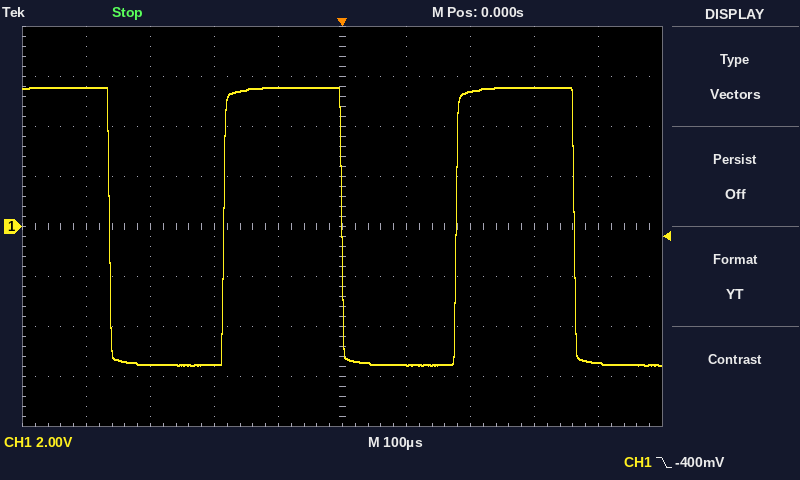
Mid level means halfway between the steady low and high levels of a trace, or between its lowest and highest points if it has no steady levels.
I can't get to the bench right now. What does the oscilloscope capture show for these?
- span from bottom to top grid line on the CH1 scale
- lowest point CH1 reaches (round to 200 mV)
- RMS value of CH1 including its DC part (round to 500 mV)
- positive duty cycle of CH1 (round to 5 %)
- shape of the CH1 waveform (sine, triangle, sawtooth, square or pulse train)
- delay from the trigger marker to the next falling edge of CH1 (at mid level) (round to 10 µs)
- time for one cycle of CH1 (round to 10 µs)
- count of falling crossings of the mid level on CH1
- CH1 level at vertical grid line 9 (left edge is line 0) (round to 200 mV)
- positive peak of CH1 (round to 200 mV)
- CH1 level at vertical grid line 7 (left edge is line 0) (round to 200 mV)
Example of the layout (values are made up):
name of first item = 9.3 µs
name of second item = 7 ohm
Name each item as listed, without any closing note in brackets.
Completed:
span from bottom to top grid line on the CH1 scale = 16 V
lowest point CH1 reaches = -5.6 V
RMS value of CH1 including its DC part = 5.5 V
positive duty cycle of CH1 = 50 %
shape of the CH1 waveform = square
delay from the trigger marker to the next falling edge of CH1 (at mid level) = 360 µs
time for one cycle of CH1 = 360 µs
count of falling crossings of the mid level on CH1 = 3
CH1 level at vertical grid line 9 (left edge is line 0) = -5.4 V
positive peak of CH1 = 5.6 V
CH1 level at vertical grid line 7 (left edge is line 0) = 5.4 V
